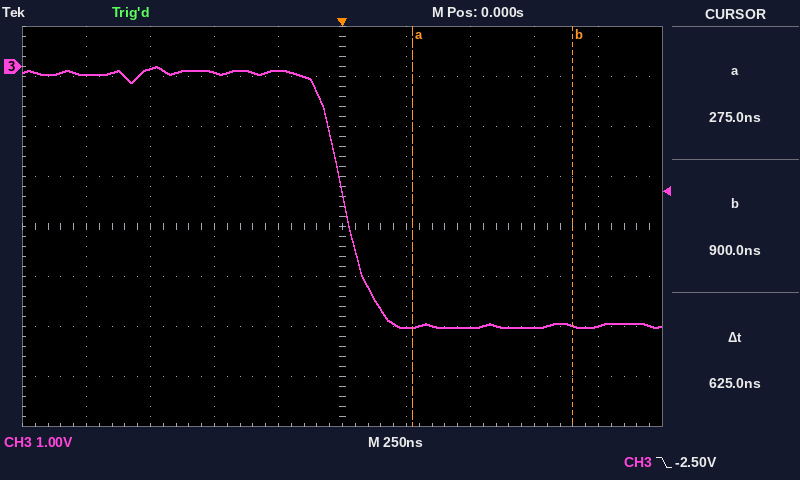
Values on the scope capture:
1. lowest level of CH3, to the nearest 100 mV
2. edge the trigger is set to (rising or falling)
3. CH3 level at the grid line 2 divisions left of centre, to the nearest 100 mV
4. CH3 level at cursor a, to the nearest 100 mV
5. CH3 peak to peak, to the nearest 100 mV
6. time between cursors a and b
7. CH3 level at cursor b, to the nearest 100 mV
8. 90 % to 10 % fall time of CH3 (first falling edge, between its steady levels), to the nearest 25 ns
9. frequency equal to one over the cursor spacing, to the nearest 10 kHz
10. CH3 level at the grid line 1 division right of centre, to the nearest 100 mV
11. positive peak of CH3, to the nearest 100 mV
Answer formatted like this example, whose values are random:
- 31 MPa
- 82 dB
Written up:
- -5.2 V
- falling
- -100 mV
- -5.2 V
- 5.2 V
- 625 ns
- -5.2 V
- 225 ns
- 1.60 MHz
- -5.2 V
- 0.0 V
